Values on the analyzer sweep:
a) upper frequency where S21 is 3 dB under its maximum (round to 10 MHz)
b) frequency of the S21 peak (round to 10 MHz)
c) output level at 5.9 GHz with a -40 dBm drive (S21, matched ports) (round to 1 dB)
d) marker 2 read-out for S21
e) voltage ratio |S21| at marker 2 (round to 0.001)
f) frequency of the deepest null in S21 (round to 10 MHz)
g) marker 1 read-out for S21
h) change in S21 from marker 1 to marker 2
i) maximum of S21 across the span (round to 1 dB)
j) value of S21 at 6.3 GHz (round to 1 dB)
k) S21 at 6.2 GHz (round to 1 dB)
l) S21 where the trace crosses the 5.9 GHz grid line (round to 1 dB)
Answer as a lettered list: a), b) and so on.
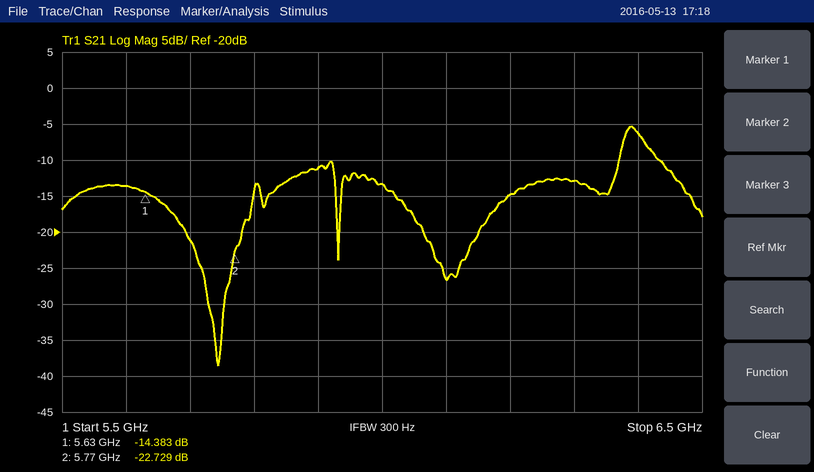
a) 6.42 GHz
b) 6.39 GHz
c) -51 dBm
d) -22.729 dB
e) 0.073
f) 5.74 GHz
g) -14.383 dB
h) -8.346 dB
i) -5 dB
j) -13 dB
k) -15 dB
l) -11 dB
